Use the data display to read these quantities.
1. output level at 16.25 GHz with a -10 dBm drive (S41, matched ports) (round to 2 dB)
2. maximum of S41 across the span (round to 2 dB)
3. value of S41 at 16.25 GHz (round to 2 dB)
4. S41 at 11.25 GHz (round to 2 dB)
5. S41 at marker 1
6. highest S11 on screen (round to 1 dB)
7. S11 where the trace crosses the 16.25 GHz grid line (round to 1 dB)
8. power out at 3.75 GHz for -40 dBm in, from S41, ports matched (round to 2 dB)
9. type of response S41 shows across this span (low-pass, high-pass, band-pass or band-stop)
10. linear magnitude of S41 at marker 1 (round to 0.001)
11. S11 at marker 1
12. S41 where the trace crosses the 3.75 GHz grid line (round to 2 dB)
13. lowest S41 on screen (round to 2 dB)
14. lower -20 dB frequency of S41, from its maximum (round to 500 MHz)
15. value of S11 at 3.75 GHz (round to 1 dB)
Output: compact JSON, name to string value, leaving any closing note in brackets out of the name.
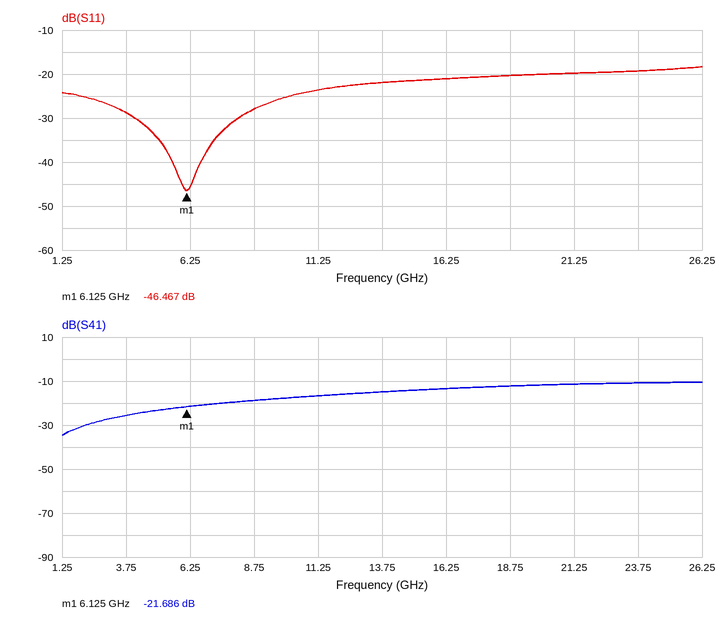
{"output level at 16.25 GHz with a -10 dBm drive (S41, matched ports)": "-24 dBm", "maximum of S41 across the span": "-10 dB", "value of S41 at 16.25 GHz": "-14 dB", "S41 at 11.25 GHz": "-16 dB", "S41 at marker 1": "-21.686 dB", "highest S11 on screen": "-18 dB", "S11 where the trace crosses the 16.25 GHz grid line": "-21 dB", "power out at 3.75 GHz for -40 dBm in, from S41, ports matched": "-66 dBm", "type of response S41 shows across this span": "high-pass", "linear magnitude of S41 at marker 1": "0.082", "S11 at marker 1": "-46.467 dB", "S41 where the trace crosses the 3.75 GHz grid line": "-26 dB", "lowest S41 on screen": "-34 dB", "lower -20 dB frequency of S41, from its maximum": "2.0 GHz", "value of S11 at 3.75 GHz": "-29 dB"}
